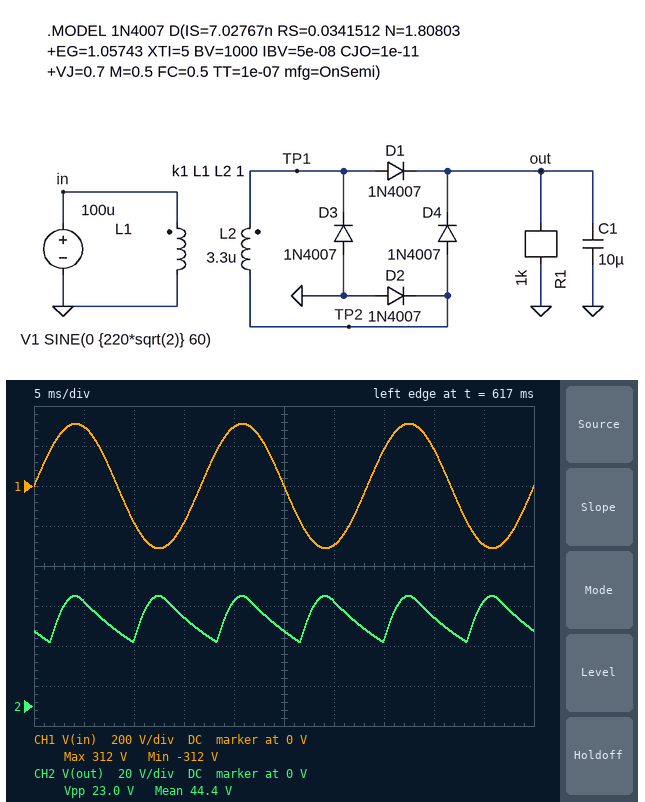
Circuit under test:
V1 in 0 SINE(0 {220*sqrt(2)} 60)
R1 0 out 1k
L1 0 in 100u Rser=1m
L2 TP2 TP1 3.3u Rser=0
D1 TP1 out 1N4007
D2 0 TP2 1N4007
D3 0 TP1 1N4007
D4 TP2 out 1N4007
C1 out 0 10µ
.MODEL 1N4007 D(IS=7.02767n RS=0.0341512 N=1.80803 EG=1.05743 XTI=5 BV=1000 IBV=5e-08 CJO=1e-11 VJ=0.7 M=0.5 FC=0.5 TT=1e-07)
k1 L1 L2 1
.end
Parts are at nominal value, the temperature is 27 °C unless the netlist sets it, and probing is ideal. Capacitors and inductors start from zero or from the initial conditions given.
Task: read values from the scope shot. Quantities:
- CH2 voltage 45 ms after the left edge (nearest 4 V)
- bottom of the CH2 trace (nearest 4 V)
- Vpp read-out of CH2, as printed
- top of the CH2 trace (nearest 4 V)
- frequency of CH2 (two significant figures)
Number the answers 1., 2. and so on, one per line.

1. 52 V
2. 32 V
3. 23.0 V
4. 56 V
5. 120 Hz
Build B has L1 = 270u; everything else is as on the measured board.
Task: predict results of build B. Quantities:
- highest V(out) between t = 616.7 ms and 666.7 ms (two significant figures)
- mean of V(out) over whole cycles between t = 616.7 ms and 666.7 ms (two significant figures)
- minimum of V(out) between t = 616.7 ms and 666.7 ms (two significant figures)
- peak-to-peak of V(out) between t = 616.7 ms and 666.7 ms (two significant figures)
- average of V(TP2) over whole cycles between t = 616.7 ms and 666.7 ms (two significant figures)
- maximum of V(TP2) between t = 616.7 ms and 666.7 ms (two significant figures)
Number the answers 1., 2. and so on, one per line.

1. 33 V
2. 27 V
3. 19 V
4. 14 V
5. 13 V
6. 34 V
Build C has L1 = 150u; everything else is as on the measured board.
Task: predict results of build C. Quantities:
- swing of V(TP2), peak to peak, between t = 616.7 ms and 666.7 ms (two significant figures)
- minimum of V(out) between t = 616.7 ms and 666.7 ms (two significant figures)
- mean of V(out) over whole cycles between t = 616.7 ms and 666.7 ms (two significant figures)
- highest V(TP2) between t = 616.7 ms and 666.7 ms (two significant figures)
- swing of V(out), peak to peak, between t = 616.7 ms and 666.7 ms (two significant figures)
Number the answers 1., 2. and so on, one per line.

1. 46 V
2. 26 V
3. 36 V
4. 45 V
5. 19 V
